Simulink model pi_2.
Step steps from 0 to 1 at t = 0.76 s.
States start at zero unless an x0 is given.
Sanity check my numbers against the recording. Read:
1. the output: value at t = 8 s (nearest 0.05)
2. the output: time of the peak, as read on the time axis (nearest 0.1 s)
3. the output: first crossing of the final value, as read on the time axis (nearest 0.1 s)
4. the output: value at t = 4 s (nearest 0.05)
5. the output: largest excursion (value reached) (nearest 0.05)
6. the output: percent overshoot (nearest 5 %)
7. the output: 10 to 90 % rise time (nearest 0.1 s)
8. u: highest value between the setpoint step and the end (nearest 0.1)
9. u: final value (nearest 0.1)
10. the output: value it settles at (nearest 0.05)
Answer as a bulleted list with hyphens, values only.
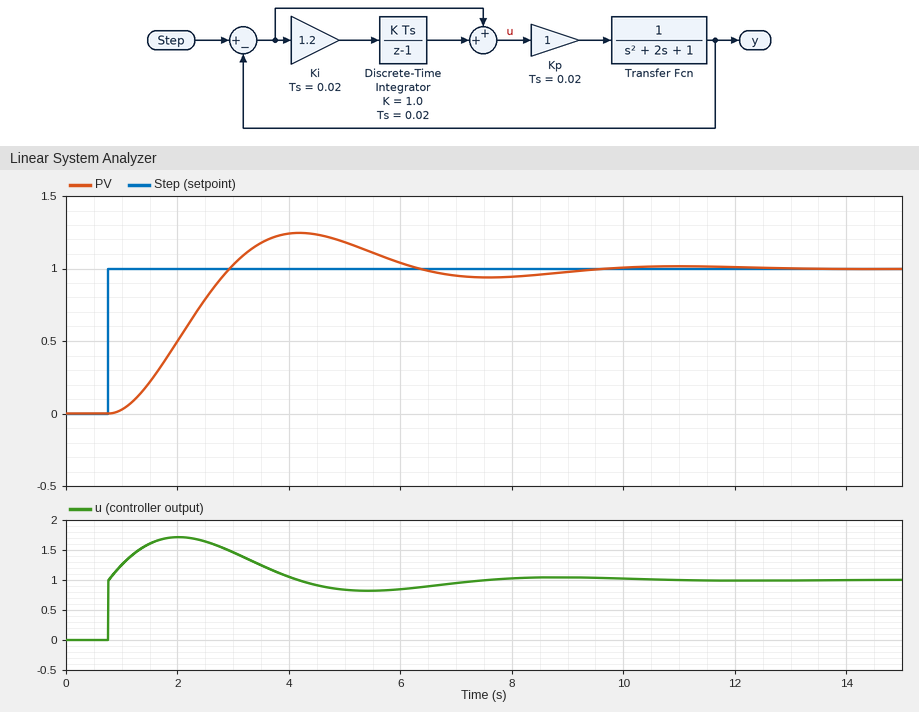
- 0.95
- 4.2 s
- 2.9 s
- 1.25
- 1.25
- 25 %
- 1.5 s
- 1.7
- 1.0
- 1.00
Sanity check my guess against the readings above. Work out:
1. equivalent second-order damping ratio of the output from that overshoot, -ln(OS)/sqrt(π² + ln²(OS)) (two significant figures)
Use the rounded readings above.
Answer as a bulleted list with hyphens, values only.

- 0.40
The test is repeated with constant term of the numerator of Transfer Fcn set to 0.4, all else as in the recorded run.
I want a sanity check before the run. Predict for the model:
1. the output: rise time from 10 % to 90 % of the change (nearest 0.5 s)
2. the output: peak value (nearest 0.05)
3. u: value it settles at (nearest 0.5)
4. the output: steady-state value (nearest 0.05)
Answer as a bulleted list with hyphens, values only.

- 3.0 s
- 1.05
- 2.5
- 1.00
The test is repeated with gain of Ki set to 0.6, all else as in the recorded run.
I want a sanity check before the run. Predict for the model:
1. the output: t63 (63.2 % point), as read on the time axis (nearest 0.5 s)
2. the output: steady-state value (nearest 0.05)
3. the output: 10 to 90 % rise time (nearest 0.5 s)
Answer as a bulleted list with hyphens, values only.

- 2.5 s
- 1.00
- 2.5 s
